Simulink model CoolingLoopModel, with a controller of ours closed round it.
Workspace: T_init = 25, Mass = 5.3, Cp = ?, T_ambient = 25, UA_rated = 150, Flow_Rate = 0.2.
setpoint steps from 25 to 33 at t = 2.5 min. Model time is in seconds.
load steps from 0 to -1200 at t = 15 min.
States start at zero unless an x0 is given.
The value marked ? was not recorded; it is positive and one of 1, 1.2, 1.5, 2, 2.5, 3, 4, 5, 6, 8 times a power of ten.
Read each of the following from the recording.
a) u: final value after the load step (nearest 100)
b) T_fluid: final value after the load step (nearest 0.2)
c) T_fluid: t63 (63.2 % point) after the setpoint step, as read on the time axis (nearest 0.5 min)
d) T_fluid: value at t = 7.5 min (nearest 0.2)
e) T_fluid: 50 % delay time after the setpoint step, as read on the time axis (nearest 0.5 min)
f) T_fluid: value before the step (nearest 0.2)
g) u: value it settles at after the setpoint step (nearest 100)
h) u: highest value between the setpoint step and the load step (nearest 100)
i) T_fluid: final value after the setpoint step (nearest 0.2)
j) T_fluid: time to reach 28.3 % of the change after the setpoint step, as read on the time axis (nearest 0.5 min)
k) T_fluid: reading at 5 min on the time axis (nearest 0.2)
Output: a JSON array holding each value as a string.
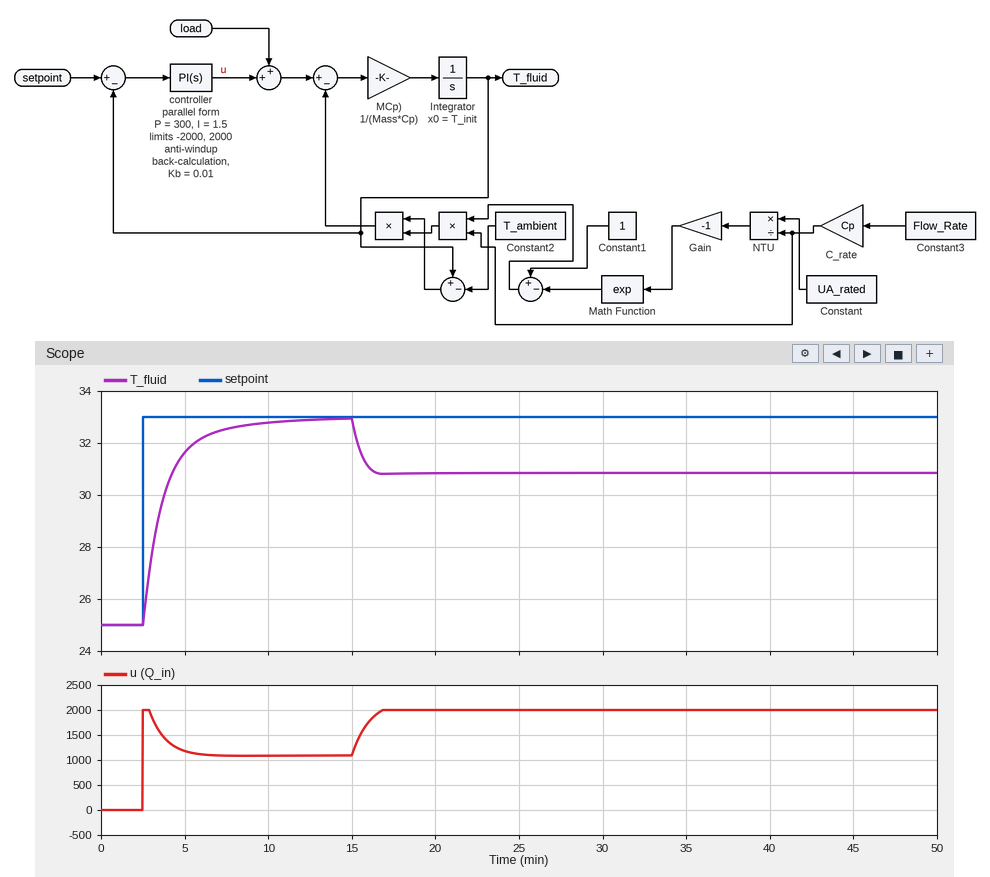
["2000", "30.8", "4.0 min", "32.6", "3.5 min", "25.0", "1100", "2000", "33.0", "3.0 min", "31.6"]
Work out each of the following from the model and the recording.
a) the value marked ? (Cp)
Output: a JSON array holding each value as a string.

["4000"]
